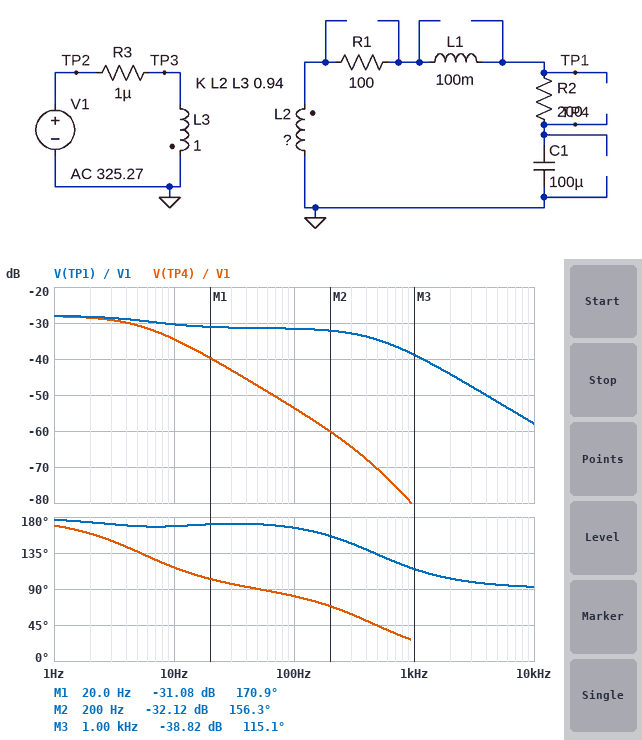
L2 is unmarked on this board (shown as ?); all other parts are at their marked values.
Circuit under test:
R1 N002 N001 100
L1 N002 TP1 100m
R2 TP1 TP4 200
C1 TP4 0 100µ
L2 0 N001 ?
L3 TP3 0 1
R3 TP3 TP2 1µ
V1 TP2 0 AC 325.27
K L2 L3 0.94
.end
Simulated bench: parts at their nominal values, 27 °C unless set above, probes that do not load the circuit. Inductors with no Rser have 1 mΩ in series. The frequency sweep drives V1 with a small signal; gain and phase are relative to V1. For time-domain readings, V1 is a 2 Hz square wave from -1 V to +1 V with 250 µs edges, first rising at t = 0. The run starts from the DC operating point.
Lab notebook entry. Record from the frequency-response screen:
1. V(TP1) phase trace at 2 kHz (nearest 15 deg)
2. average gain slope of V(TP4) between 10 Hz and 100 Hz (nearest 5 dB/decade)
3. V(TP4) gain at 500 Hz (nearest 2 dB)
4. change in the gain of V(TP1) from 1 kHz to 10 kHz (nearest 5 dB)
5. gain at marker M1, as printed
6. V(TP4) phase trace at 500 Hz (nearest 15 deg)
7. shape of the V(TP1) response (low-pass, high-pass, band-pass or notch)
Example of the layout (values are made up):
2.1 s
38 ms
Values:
105 deg
-20 dB/decade
-70 dB
-20 dB
-31.08 dB
45 deg
low-pass
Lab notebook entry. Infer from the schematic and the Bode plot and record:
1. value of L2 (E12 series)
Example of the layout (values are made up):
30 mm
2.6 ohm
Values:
1.8 mH
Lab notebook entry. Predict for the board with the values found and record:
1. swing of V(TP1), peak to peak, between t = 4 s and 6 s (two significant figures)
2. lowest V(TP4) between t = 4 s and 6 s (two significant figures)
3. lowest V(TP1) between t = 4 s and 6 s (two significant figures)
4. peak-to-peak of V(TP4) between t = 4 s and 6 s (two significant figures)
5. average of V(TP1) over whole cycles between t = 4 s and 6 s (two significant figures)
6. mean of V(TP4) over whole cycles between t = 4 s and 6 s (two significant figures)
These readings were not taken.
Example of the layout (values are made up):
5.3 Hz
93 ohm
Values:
80 mV
-80 mV
-80 mV
80 mV
-40 mV
-40 mV
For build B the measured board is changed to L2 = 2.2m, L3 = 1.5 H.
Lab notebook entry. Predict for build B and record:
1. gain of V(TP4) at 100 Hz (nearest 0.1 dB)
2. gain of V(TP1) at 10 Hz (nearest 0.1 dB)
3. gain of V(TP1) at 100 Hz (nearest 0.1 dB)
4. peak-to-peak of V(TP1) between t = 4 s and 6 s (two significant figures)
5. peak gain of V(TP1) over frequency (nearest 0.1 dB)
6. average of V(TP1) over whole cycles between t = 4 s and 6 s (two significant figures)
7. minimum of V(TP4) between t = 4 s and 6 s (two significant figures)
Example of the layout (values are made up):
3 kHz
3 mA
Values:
-54.5 dB
-31.3 dB
-32.5 dB
72 mV
-28.9 dB
-36 mV
-72 mV
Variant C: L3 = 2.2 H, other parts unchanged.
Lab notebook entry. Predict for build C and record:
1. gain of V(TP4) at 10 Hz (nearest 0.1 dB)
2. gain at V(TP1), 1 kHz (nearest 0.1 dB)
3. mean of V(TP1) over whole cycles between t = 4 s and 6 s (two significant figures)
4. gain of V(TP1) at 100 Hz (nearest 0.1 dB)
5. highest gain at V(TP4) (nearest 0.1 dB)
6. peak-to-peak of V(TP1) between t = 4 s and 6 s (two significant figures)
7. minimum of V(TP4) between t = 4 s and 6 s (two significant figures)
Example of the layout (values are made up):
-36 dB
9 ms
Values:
-37.9 dB
-42.2 dB
-27 mV
-35.0 dB
-31.4 dB
54 mV
-54 mV
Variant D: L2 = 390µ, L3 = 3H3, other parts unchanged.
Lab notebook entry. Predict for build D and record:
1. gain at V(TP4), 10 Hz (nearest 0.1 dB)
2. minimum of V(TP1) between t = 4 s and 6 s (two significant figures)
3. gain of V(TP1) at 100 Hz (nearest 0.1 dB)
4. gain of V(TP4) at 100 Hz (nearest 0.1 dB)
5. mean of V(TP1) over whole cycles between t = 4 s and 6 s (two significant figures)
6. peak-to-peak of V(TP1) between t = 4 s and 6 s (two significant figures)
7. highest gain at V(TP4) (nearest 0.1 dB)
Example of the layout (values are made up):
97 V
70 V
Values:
-46.3 dB
-20 mV
-43.4 dB
-65.4 dB
-10 mV
20 mV
-39.8 dB
